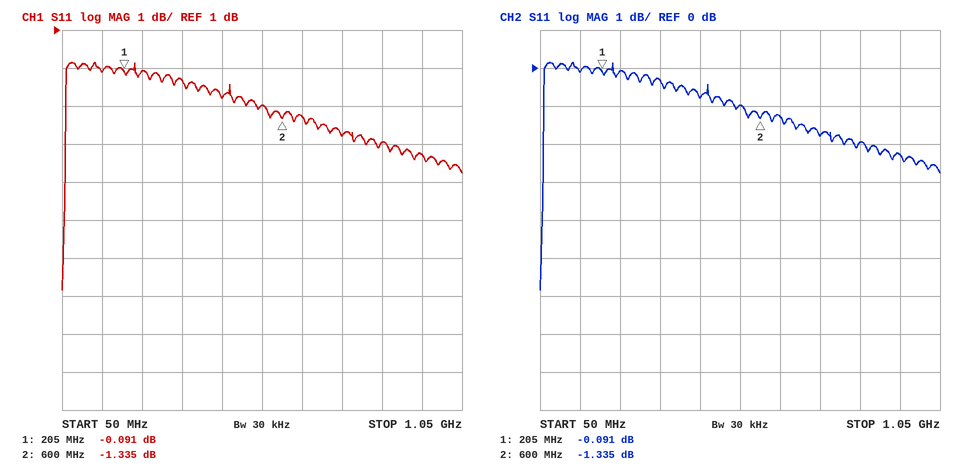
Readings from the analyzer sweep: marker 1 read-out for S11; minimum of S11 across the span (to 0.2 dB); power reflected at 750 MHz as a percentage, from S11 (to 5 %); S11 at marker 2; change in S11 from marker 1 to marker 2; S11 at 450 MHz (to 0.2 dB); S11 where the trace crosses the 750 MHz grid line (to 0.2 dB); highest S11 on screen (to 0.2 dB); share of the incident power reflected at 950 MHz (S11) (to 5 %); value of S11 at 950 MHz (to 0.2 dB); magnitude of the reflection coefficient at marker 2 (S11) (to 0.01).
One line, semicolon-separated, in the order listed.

-0.091 dB; -5.8 dB; 65 %; -1.335 dB; -1.244 dB; -0.8 dB; -1.8 dB; 0.2 dB; 60 %; -2.2 dB; 0.86
